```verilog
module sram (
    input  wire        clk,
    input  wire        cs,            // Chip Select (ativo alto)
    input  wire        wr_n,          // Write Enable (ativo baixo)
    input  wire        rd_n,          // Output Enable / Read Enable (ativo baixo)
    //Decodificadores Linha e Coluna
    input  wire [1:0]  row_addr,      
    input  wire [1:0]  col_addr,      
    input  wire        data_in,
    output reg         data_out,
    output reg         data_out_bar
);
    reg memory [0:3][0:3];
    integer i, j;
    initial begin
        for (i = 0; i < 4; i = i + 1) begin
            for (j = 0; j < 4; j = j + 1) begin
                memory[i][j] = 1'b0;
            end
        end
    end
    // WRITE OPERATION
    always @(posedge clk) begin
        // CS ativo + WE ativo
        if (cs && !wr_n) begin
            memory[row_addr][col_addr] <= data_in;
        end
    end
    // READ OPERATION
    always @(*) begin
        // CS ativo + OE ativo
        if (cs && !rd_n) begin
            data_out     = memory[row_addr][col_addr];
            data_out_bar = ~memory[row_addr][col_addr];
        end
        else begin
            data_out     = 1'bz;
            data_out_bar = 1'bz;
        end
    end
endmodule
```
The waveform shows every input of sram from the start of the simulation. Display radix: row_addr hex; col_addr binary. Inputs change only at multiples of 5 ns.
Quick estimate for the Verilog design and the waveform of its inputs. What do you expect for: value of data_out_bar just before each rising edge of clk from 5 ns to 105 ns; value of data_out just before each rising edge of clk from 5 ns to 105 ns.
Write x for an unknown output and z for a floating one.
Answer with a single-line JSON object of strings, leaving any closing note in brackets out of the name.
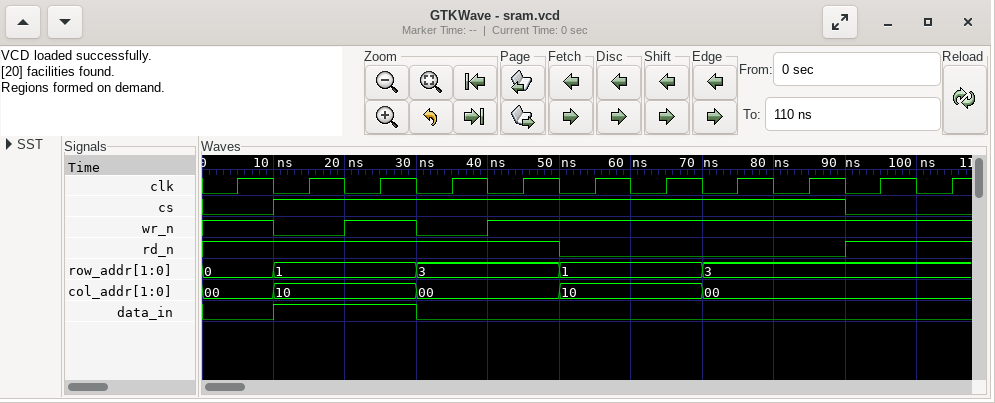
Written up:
{"value of data_out_bar just before each rising edge of clk from 5 ns to 105 ns": "z z z z z 0 0 1 1 z z", "value of data_out just before each rising edge of clk from 5 ns to 105 ns": "z z z z z 1 1 0 0 z z"}
